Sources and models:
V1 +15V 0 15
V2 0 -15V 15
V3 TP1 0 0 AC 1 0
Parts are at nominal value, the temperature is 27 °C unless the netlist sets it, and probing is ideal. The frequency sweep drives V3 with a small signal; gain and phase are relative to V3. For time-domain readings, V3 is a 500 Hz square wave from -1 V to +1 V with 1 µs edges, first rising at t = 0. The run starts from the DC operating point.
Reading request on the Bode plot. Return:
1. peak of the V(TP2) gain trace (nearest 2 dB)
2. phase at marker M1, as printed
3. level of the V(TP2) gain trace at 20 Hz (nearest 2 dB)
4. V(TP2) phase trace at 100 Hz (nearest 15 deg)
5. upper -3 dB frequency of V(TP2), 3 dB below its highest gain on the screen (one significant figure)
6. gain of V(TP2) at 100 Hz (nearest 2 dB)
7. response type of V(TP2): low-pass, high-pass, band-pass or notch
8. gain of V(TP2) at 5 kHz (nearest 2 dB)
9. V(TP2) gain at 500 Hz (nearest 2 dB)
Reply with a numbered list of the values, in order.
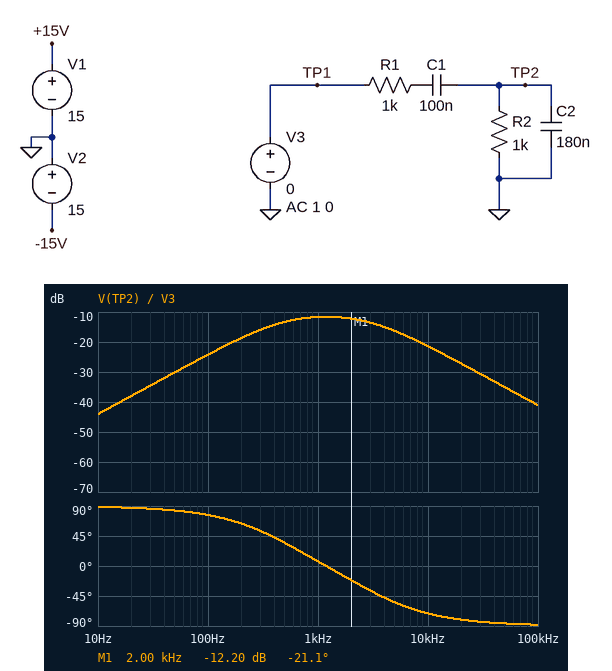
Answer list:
1. -12 dB
2. -21.1 deg
3. -38 dB
4. 75 deg
5. 4 kHz
6. -24 dB
7. band-pass
8. -16 dB
9. -14 dB
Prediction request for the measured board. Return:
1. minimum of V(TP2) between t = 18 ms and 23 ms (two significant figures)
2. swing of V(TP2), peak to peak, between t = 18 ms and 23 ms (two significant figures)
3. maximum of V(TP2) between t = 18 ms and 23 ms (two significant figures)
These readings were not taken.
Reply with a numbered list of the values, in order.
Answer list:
1. -410 mV
2. 810 mV
3. 410 mV
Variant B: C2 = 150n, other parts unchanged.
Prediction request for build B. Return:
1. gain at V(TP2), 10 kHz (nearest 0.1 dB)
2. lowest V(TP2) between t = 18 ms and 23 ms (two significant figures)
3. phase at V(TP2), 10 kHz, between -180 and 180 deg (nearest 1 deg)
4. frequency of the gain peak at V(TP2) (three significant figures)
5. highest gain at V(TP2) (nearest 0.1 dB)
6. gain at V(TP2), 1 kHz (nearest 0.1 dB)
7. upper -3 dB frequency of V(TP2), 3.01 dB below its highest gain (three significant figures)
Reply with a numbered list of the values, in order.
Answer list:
1. -19.9 dB
2. -450 mV
3. -69 deg
4. 1.30 kHz
5. -10.9 dB
6. -11.0 dB
7. 4.12 kHz
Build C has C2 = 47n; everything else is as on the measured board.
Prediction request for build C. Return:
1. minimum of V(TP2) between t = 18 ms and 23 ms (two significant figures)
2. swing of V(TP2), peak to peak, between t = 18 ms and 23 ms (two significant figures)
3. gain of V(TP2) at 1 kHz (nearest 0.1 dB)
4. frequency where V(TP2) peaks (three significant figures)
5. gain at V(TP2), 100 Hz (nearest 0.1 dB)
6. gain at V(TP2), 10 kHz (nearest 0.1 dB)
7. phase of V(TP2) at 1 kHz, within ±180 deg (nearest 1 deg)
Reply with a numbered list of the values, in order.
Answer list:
1. -690 mV
2. 1.4 V
3. -8.9 dB
4. 2.32 kHz
5. -24.1 dB
6. -11.4 dB
7. 28 deg
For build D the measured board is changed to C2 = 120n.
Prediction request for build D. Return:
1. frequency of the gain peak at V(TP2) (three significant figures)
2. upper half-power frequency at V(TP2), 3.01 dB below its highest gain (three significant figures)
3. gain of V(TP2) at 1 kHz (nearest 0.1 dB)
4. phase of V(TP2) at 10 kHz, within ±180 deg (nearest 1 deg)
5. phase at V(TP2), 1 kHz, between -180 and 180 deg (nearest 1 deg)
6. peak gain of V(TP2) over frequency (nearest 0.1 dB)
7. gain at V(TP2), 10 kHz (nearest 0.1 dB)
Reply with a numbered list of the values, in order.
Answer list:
1. 1.45 kHz
2. 4.69 kHz
3. -10.4 dB
4. -67 deg
5. 15 deg
6. -10.1 dB
7. -18.1 dB
